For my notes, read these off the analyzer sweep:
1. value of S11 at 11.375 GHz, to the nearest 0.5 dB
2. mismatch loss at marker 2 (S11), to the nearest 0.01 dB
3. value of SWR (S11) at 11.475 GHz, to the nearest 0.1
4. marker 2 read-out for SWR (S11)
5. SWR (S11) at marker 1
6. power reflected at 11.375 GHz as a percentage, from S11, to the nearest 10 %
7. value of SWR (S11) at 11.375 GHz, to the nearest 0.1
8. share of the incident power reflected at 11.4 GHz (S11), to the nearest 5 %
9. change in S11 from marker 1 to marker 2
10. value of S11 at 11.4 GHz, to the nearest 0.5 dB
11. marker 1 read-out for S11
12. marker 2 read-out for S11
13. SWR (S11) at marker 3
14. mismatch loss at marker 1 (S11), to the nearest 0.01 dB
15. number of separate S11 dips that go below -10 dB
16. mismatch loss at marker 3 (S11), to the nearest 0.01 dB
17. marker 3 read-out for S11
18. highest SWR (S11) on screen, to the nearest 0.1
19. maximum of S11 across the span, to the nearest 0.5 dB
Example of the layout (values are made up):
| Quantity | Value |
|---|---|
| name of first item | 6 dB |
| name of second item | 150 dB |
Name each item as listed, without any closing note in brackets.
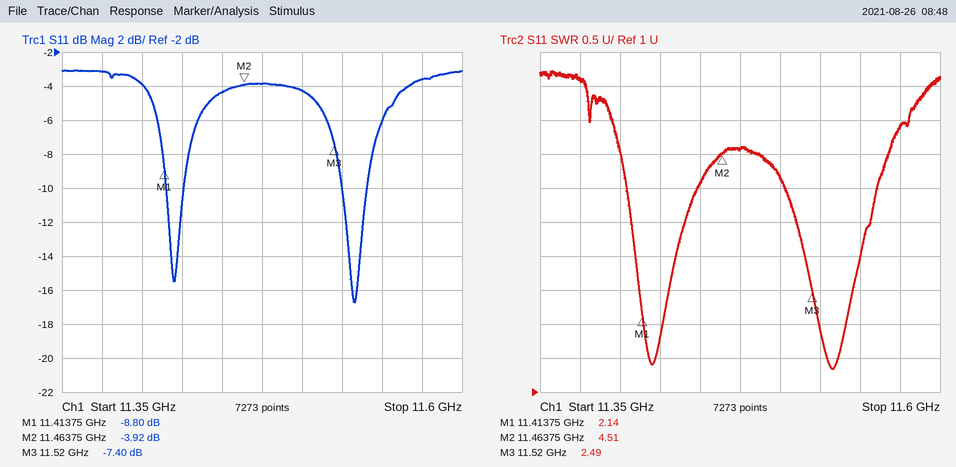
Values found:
| Quantity | Value |
|---|---|
| value of S11 at 11.375 GHz, to the nearest 0.5 dB | -3.0 dB |
| mismatch loss at marker 2 (S11), to the nearest 0.01 dB | 2.26 dB |
| value of SWR (S11) at 11.475 GHz, to the nearest 0.1 | 4.6 |
| marker 2 read-out for SWR | 4.51 |
| SWR (S11) at marker 1 | 2.14 |
| power reflected at 11.375 GHz as a percentage, from S11, to the nearest 10 % | 50 % |
| value of SWR (S11) at 11.375 GHz, to the nearest 0.1 | 5.6 |
| share of the incident power reflected at 11.4 GHz (S11), to the nearest 5 % | 40 % |
| change in S11 from marker 1 to marker 2 | 4.88 dB |
| value of S11 at 11.4 GHz, to the nearest 0.5 dB | -4.0 dB |
| marker 1 read-out for S11 | -8.80 dB |
| marker 2 read-out for S11 | -3.92 dB |
| SWR (S11) at marker 3 | 2.49 |
| mismatch loss at marker 1 (S11), to the nearest 0.01 dB | 0.61 dB |
| number of separate S11 dips that go below -10 dB | 2 |
| mismatch loss at marker 3 (S11), to the nearest 0.01 dB | 0.87 dB |
| marker 3 read-out for S11 | -7.40 dB |
| highest SWR (S11) on screen, to the nearest 0.1 | 5.7 |
| maximum of S11 across the span, to the nearest 0.5 dB | -3.0 dB |
